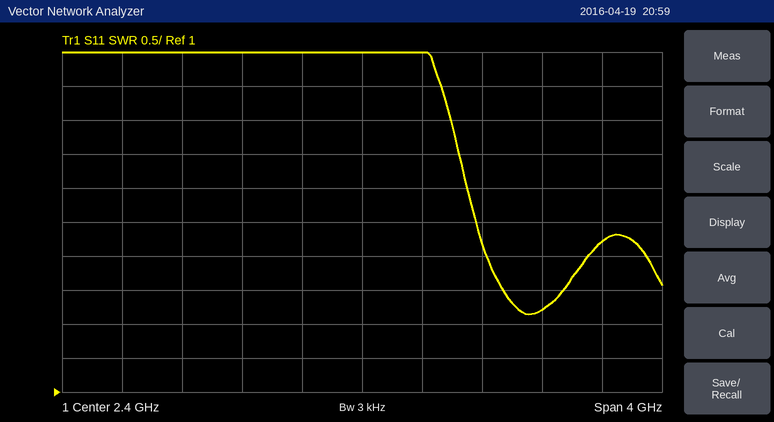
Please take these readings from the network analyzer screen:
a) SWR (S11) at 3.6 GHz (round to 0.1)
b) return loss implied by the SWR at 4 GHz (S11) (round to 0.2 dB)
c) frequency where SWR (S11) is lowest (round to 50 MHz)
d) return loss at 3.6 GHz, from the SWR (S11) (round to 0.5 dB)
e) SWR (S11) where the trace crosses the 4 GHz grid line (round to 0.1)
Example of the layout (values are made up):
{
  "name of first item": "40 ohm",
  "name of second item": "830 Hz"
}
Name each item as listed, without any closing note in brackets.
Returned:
{
  "SWR (S11) at 3.6 GHz": "2.2",
  "return loss implied by the SWR at 4 GHz (S11)": "5.6 dB",
  "frequency where SWR (S11) is lowest": "3.50 GHz",
  "return loss at 3.6 GHz, from the SWR (S11)": "8.5 dB",
  "SWR (S11) where the trace crosses the 4 GHz grid line": "3.2"
}
